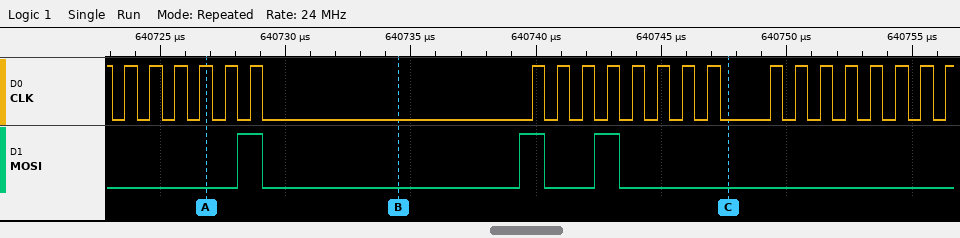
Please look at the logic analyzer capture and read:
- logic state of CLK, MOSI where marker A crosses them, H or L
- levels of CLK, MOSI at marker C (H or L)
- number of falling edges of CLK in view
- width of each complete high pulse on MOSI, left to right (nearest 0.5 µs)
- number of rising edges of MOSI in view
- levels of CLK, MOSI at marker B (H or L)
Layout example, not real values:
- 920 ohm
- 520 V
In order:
- CLK=H, MOSI=L
- CLK=L, MOSI=L
- 22
- 1 µs, 1 µs, 1 µs
- 3
- CLK=L, MOSI=L
